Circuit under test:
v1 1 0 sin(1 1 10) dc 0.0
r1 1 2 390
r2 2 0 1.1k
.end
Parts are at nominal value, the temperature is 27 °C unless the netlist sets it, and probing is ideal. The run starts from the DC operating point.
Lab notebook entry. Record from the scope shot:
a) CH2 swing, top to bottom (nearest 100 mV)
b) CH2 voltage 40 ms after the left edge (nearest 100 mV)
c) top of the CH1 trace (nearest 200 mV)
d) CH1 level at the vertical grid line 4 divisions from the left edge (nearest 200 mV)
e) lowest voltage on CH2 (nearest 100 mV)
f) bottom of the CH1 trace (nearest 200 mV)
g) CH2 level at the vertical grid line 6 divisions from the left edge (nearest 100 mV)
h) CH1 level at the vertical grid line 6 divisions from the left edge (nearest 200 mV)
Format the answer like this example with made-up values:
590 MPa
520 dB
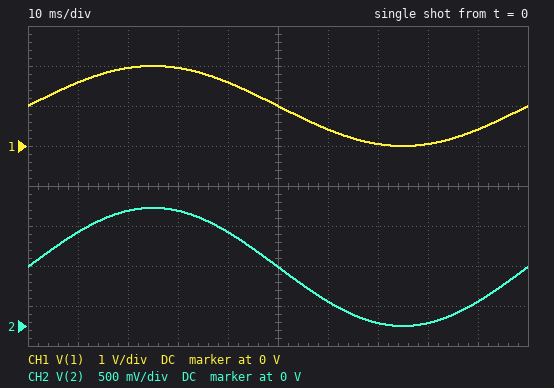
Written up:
1.5 V
1.2 V
2.0 V
1.6 V
0 V
0 V
300 mV
400 mV
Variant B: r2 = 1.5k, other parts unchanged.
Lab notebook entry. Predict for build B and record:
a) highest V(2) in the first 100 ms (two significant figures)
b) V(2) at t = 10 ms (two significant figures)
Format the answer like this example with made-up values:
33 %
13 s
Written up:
1.6 V
1.3 V
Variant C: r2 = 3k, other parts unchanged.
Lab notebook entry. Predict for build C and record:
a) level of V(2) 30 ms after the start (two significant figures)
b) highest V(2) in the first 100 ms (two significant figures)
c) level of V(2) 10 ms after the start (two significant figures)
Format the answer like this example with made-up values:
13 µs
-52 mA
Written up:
1.7 V
1.8 V
1.4 V
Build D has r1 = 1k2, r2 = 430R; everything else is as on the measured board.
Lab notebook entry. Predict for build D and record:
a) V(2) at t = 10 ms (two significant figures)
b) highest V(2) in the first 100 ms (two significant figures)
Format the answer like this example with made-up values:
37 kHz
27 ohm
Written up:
420 mV
530 mV
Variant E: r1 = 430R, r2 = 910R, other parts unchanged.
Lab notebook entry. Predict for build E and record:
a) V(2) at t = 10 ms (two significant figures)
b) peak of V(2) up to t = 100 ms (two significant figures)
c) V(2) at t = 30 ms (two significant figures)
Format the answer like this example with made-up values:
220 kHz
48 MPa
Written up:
1.1 V
1.4 V
1.3 V
